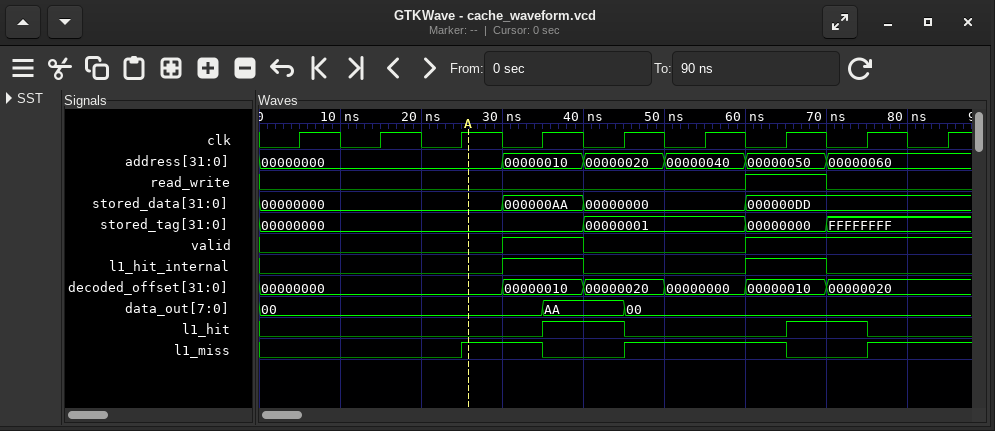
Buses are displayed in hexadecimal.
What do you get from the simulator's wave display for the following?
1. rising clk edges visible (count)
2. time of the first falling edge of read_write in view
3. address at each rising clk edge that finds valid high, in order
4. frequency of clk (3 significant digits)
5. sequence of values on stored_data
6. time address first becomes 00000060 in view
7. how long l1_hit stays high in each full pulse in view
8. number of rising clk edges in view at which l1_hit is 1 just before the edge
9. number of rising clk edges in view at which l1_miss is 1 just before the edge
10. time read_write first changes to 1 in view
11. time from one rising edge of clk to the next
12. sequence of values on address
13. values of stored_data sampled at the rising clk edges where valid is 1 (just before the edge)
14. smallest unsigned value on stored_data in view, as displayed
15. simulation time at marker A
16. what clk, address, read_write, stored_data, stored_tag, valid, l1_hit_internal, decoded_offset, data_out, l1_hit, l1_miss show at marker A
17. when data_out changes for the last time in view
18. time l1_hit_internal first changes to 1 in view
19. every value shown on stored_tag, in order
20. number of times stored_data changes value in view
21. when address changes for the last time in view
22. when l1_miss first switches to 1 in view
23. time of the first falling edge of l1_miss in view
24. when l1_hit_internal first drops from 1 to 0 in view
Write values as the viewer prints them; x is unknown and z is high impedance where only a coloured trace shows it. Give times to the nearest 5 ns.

9
70 ns
00000010, 00000050, 00000060, 00000060
100 MHz
00000000, 000000AA, 00000000, 000000DD
70 ns
10 ns, 10 ns
2
4
60 ns
10 ns
00000000, 00000010, 00000020, 00000040, 00000050, 00000060
000000AA, 000000DD, 000000DD, 000000DD
00000000
25 ns
clk=1, address=00000000, read_write=0, stored_data=00000000, stored_tag=00000000, valid=0, l1_hit_internal=0, decoded_offset=00000000, data_out=00, l1_hit=0, l1_miss=1
45 ns
30 ns
00000000, 00000001, 00000000, FFFFFFFF
3
70 ns
25 ns
35 ns
40 ns
